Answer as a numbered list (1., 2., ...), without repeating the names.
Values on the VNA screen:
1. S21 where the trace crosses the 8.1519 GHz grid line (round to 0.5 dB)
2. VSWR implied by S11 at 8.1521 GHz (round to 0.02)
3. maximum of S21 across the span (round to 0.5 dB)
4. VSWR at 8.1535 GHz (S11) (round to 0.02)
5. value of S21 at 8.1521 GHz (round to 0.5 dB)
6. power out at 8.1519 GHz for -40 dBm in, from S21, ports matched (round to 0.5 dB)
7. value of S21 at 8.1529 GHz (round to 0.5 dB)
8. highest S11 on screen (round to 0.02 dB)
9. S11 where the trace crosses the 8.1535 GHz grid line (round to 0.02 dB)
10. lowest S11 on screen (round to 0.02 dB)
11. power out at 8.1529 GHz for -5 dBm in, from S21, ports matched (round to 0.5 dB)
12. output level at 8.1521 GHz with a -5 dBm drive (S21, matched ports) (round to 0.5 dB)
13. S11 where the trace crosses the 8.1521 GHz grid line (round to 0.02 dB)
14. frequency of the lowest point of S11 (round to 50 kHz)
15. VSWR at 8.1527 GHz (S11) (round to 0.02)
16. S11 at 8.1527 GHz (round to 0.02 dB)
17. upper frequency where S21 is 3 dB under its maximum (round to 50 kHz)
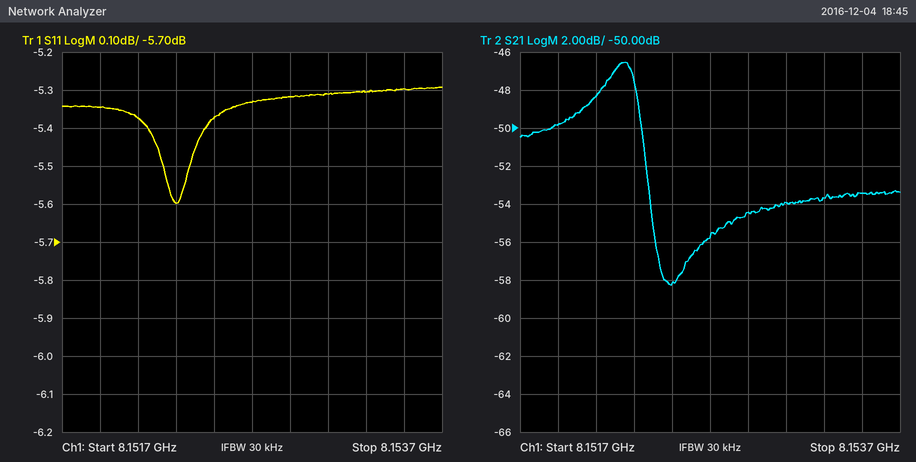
1. -50.0 dB
2. 3.34
3. -46.5 dB
4. 3.38
5. -48.5 dB
6. -90.0 dBm
7. -54.5 dB
8. -5.30 dB
9. -5.30 dB
10. -5.60 dB
11. -59.5 dBm
12. -53.5 dBm
13. -5.38 dB
14. 8.15230 GHz
15. 3.36
16. -5.34 dB
17. 8.15235 GHz
